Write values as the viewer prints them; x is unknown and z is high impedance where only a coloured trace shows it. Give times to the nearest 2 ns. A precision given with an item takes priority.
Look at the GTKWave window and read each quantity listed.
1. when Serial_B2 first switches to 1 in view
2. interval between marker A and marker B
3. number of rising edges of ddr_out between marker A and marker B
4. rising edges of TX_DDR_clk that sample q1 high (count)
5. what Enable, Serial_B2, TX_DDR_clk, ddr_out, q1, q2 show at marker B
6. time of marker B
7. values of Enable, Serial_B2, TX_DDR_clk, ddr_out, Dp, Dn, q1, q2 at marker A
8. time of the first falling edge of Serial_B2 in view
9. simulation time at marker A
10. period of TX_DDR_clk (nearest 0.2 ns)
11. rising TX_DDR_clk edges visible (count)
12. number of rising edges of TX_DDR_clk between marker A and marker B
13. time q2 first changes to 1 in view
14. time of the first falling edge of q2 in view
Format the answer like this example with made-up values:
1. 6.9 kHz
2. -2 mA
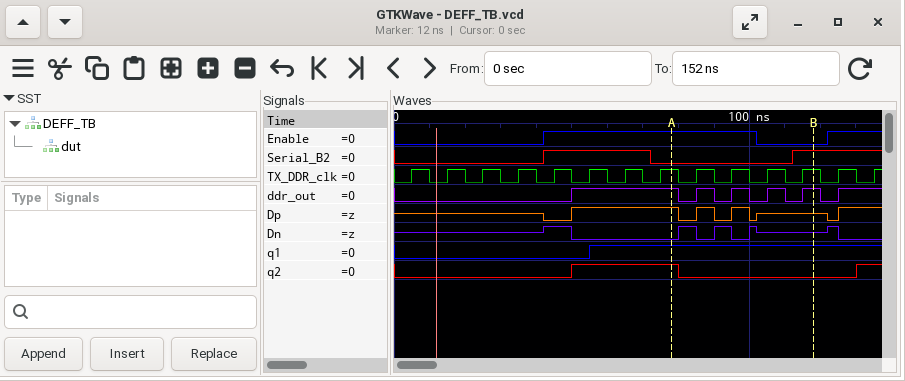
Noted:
1. 42 ns
2. 40 ns
3. 4
4. 8
5. Enable=0, Serial_B2=1, TX_DDR_clk=1, ddr_out=1, q1=1, q2=0
6. 118 ns
7. Enable=1, Serial_B2=0, TX_DDR_clk=1, ddr_out=1, Dp=1, Dn=0, q1=1, q2=1
8. 72 ns
9. 78 ns
10. 10 ns
11. 14
12. 4
13. 50 ns
14. 80 ns
